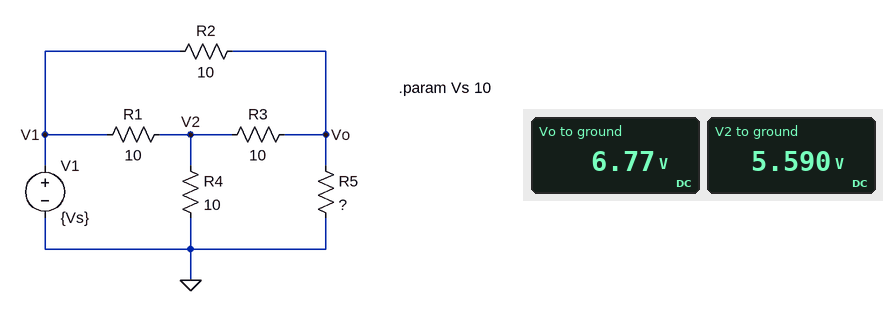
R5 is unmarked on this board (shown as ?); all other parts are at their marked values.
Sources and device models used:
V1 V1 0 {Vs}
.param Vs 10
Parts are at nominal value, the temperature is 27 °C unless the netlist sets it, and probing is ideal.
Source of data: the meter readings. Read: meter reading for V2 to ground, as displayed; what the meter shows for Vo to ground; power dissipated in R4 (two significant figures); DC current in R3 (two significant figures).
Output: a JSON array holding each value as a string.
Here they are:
["5.590 V", "6.77 V", "3.1 W", "120 mA"]
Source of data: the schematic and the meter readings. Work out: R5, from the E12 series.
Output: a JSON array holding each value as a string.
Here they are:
["33 Ω"]
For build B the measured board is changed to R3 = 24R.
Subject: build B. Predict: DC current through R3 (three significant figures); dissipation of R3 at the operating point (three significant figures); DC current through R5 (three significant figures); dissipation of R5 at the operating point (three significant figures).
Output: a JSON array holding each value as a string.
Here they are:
["72.9 mA", "128 mW", "216 mA", "1.53 W"]
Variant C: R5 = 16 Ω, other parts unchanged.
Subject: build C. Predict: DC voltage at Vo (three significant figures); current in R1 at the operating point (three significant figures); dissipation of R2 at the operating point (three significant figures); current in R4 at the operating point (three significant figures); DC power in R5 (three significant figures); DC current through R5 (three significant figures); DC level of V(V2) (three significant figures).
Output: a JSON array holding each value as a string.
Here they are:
["5.82 V", "473 mA", "1.75 W", "527 mA", "2.12 W", "364 mA", "5.27 V"]
